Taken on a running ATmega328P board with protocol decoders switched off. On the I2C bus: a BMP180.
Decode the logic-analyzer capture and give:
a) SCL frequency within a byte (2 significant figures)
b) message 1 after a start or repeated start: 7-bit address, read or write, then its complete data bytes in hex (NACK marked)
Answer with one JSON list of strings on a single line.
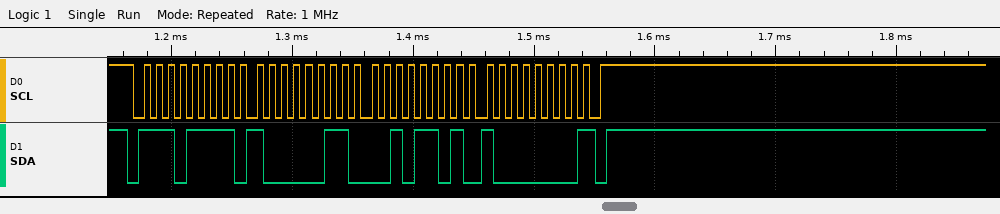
["100 kHz", "0x77 read: 83 2D 80 NACK"]
